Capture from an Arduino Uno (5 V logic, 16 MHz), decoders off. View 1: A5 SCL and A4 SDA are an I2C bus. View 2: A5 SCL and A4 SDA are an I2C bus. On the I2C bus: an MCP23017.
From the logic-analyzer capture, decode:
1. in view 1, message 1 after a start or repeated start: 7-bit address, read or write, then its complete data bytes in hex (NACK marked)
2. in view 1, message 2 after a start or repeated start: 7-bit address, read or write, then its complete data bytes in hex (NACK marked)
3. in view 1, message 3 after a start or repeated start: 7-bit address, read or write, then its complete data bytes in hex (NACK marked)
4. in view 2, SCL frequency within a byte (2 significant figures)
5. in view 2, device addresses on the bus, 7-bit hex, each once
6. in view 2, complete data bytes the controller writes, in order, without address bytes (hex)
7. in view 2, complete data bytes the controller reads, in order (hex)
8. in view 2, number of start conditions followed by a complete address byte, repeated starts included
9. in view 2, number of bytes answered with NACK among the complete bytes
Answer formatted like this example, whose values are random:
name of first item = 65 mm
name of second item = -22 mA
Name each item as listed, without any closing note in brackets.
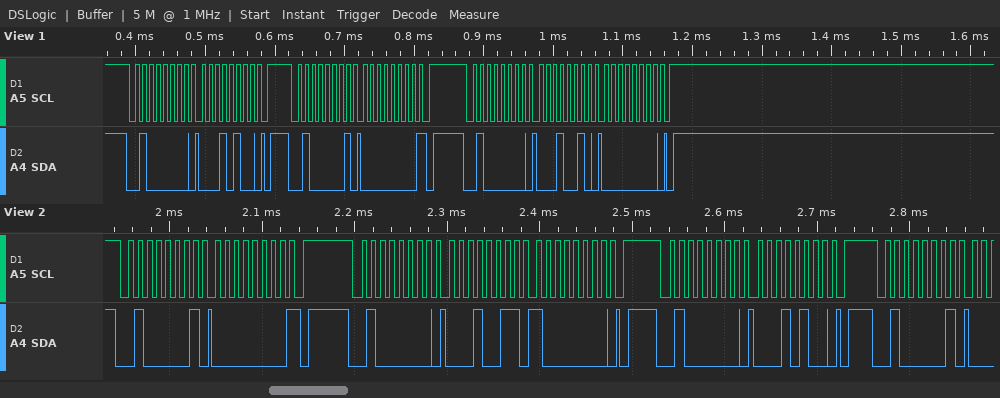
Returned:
in view 1, message 1 after a start or repeated start: 7-bit address, read or write, then its complete data bytes in hex = 0x20 write: 14
in view 1, message 2 after a start or repeated start: 7-bit address, read or write, then its complete data bytes in hex = 0x20 read: 00 NACK
in view 1, message 3 after a start or repeated start: 7-bit address, read or write, then its complete data bytes in hex = 0x20 write: 12 00
in view 2, SCL frequency within a byte = 100 kHz
in view 2, device addresses on the bus, 7-bit hex, each once = 0x20
in view 2, complete data bytes the controller writes, in order, without address bytes = 13 80 14
in view 2, complete data bytes the controller reads, in order = 00
in view 2, number of start conditions followed by a complete address byte, repeated starts included = 4
in view 2, number of bytes answered with NACK among the complete bytes = 1
